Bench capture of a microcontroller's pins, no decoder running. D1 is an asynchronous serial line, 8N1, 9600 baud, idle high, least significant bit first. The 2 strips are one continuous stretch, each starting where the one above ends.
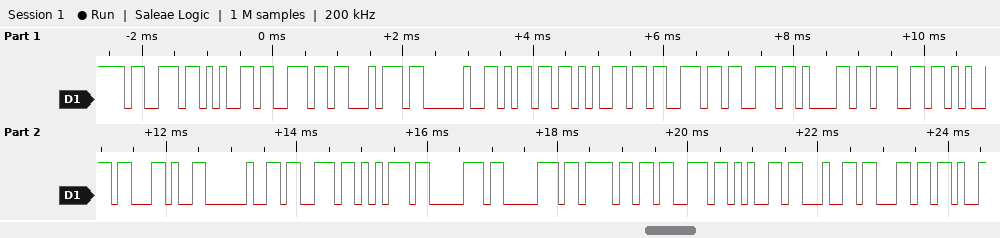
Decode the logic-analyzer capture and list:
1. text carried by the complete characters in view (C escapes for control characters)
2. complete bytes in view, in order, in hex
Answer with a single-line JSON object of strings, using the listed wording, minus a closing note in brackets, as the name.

{"text carried by the complete characters in view": "\"sent message, supposedl\"", "complete bytes in view, in order, in hex": "73 65 6E 74 20 6D 65 73 73 61 67 65 2C 20 73 75 70 70 6F 73 65 64 6C"}
